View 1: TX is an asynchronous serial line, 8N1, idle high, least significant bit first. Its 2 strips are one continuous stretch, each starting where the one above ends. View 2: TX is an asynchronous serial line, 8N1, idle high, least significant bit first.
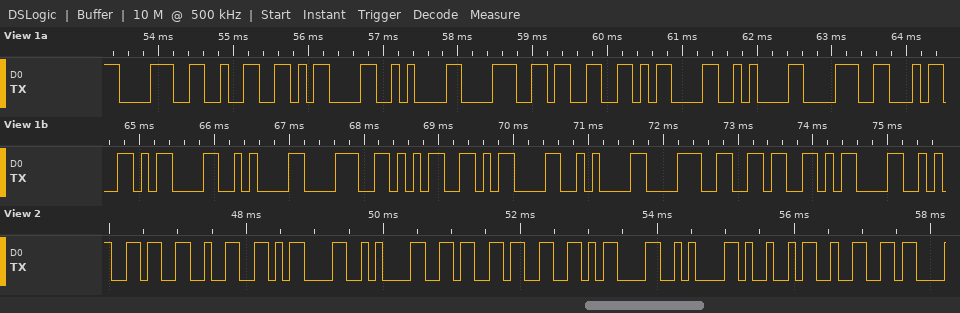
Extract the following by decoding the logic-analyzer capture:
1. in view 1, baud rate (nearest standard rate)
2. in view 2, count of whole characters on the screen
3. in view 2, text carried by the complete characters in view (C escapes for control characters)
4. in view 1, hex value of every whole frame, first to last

9600 baud
10
"62\r\n63\r\nI2"
38 32 0D 0A 38 33 0D 0A 38 34 0D 0A 38 35 0D 0A 38 36 0D
